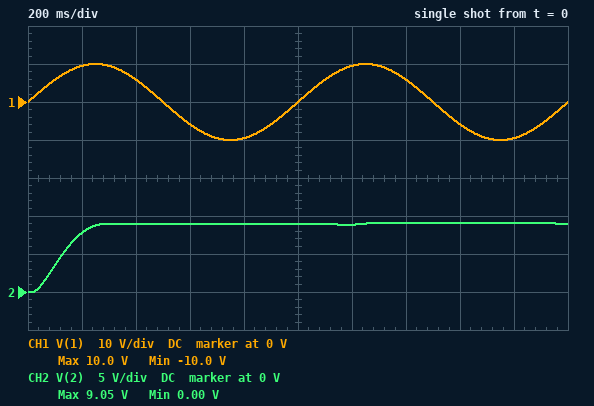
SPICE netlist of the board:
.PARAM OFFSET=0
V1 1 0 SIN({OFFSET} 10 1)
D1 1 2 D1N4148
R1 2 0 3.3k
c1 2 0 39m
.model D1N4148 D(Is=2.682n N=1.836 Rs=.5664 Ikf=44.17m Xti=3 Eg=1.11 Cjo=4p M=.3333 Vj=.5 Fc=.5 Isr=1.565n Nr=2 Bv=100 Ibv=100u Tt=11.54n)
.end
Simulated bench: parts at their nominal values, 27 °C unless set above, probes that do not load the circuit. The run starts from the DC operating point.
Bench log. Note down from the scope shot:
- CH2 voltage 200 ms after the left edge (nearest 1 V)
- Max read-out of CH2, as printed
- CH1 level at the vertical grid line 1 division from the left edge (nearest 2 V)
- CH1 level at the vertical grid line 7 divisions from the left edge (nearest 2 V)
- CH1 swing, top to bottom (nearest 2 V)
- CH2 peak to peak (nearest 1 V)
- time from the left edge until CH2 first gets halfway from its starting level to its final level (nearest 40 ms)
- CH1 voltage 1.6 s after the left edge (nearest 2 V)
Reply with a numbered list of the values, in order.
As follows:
1. 8 V
2. 9.05 V
3. 10 V
4. 6 V
5. 20 V
6. 9 V
7. 120 ms
8. -6 V
